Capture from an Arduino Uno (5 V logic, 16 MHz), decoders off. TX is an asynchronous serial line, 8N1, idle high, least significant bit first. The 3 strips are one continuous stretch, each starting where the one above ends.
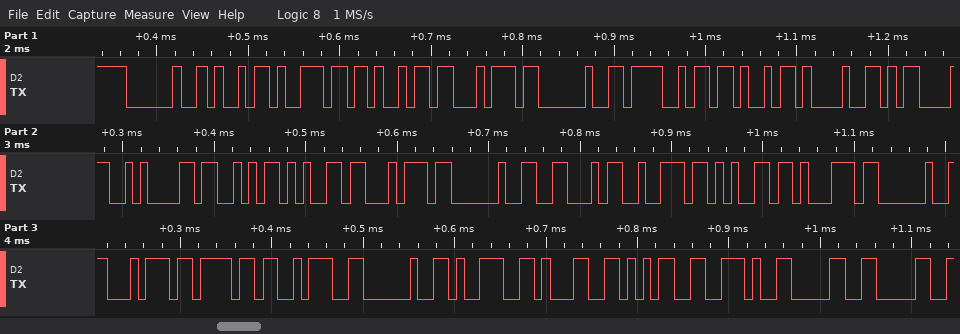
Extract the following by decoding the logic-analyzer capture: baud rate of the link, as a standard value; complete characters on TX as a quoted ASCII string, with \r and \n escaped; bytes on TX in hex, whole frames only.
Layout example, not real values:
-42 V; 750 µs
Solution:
115200 baud; " init OK!\r\nSet Freq to: 915.00"; 20 69 6E 69 74 20 4F 4B 21 0D 0A 53 65 74 20 46 72 65 71 20 74 6F 3A 20 39 31 35 2E 30 30
